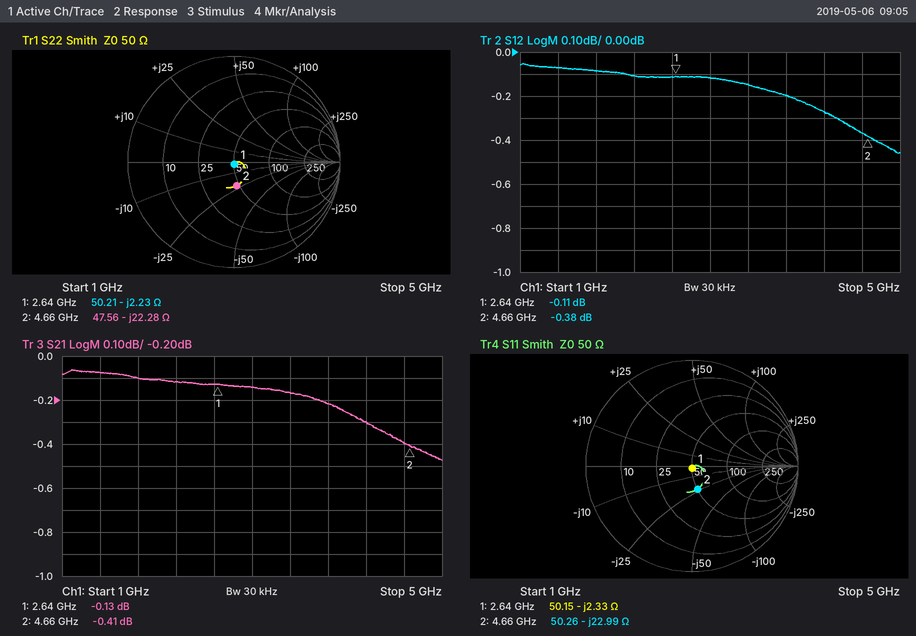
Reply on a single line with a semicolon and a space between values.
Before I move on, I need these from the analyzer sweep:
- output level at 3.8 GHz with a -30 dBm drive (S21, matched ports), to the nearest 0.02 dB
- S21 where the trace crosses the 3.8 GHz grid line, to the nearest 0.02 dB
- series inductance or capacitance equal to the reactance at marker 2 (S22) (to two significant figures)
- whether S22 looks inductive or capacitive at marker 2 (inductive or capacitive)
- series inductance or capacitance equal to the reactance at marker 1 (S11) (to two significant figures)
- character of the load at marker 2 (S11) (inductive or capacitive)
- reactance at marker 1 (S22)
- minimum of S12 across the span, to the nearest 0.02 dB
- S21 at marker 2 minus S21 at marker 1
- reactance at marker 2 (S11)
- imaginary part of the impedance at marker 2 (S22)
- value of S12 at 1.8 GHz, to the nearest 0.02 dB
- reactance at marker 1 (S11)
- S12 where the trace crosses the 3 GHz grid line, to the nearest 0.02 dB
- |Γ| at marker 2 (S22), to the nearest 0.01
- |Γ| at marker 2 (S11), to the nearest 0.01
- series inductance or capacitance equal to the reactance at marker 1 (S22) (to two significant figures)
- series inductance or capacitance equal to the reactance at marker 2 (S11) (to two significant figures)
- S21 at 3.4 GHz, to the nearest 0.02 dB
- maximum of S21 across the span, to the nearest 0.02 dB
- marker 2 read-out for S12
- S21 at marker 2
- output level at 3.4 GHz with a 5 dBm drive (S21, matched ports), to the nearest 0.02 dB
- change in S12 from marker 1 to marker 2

-30.22 dBm; -0.22 dB; 1.5 pF; capacitive; 26 pF; capacitive; -2.23 Ω; -0.46 dB; -0.28 dB; -22.99 Ω; -22.28 Ω; -0.08 dB; -2.33 Ω; -0.12 dB; 0.22; 0.22; 27 pF; 1.5 pF; -0.16 dB; -0.06 dB; -0.38 dB; -0.41 dB; 4.84 dBm; -0.27 dB
